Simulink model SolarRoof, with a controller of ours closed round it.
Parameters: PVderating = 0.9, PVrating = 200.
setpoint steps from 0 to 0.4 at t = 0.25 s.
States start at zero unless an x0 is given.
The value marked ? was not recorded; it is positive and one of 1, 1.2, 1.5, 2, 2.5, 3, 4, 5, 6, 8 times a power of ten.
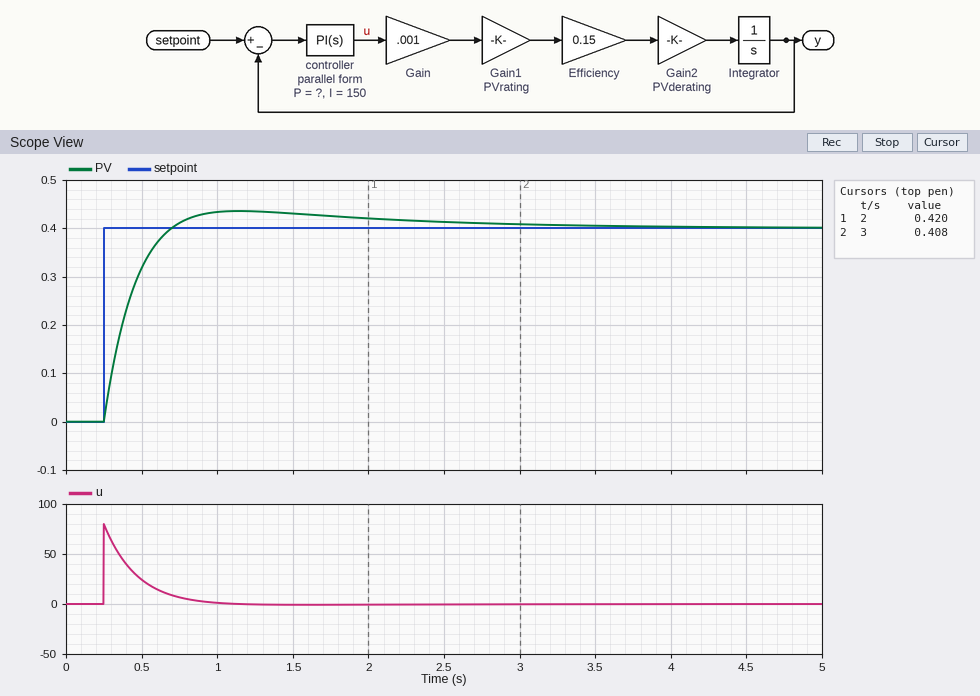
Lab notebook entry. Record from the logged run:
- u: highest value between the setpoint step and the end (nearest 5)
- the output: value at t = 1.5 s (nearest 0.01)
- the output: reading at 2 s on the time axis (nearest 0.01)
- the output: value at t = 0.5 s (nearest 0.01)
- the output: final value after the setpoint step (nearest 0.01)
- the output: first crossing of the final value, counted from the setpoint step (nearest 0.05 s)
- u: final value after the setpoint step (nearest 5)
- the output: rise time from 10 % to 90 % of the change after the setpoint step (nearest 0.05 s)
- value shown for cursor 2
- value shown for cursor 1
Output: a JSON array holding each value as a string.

["80", "0.43", "0.42", "0.32", "0.40", "0.45 s", "0", "0.30 s", "0.408", "0.420"]
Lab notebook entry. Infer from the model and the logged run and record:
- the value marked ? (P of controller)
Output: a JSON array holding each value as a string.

["200"]
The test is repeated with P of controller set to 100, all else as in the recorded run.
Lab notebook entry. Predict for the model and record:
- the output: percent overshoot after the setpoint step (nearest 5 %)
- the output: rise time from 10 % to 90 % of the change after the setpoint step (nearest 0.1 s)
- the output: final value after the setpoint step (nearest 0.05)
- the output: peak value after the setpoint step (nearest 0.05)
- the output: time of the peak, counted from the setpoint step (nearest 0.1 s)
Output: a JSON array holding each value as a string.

["20 %", "0.4 s", "0.40", "0.50", "1.1 s"]
